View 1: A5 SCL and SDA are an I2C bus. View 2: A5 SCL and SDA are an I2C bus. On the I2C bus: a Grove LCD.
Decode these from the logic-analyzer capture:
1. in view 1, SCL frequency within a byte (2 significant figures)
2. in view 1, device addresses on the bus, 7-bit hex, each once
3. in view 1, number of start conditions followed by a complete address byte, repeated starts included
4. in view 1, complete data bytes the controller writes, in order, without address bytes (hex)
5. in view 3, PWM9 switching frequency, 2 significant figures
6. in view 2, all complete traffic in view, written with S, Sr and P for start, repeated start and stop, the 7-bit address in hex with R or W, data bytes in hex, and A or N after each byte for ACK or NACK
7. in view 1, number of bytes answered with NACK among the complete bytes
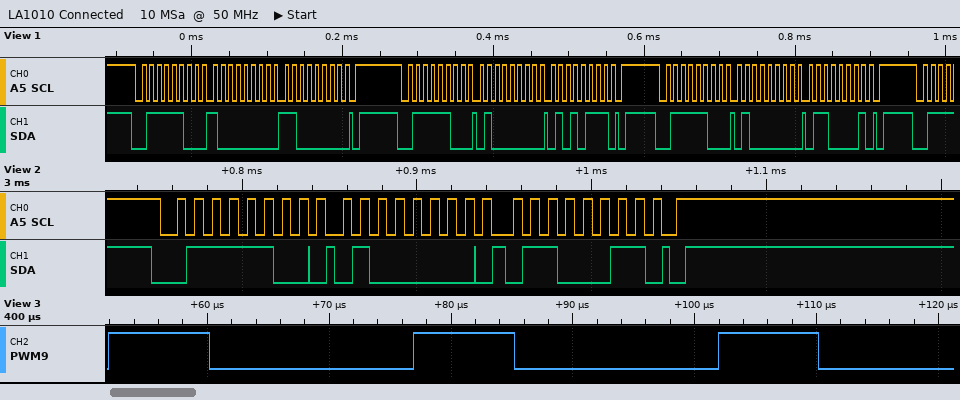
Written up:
100 kHz
0x3E
3
80 C0 40 57 40 61
40 kHz
S 3EW A 40 A 63 A P
0
